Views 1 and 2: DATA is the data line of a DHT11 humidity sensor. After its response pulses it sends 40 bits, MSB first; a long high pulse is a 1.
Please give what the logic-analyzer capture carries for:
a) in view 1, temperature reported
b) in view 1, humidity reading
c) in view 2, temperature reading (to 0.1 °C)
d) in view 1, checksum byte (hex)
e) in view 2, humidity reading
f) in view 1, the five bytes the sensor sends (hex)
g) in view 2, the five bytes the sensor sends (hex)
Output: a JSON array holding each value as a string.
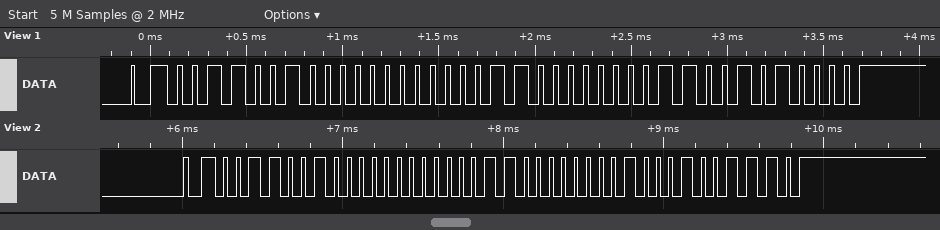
["24.6 °C", "50 %", "24.4 °C", "0x50", "50 %", "32 00 18 06 50", "32 00 18 04 4E"]
